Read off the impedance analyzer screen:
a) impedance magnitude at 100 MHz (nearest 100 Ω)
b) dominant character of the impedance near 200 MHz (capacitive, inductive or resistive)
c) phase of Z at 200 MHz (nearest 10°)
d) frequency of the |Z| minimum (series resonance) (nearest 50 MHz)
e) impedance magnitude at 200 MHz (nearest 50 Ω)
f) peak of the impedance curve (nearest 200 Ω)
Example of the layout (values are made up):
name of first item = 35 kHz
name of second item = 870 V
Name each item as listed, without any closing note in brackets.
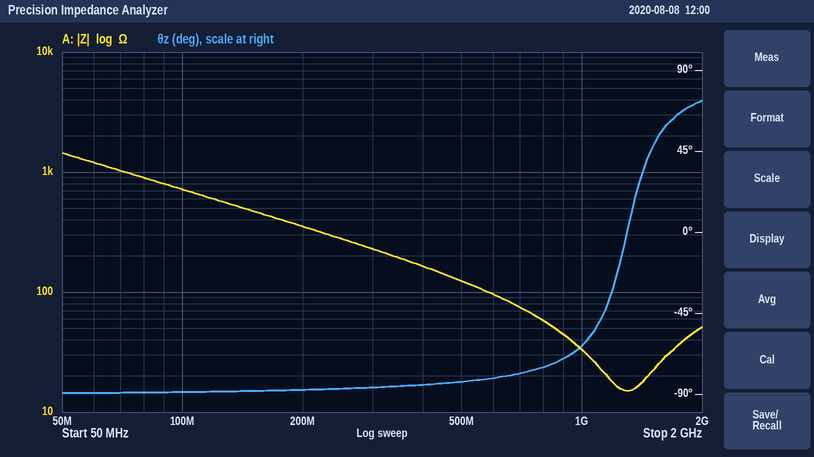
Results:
impedance magnitude at 100 MHz = 700 Ω
dominant character of the impedance near 200 MHz = capacitive
phase of Z at 200 MHz = -90°
frequency of the |Z| minimum (series resonance) = 1.30 GHz
impedance magnitude at 200 MHz = 350 Ω
peak of the impedance curve = 1.4 kΩ
